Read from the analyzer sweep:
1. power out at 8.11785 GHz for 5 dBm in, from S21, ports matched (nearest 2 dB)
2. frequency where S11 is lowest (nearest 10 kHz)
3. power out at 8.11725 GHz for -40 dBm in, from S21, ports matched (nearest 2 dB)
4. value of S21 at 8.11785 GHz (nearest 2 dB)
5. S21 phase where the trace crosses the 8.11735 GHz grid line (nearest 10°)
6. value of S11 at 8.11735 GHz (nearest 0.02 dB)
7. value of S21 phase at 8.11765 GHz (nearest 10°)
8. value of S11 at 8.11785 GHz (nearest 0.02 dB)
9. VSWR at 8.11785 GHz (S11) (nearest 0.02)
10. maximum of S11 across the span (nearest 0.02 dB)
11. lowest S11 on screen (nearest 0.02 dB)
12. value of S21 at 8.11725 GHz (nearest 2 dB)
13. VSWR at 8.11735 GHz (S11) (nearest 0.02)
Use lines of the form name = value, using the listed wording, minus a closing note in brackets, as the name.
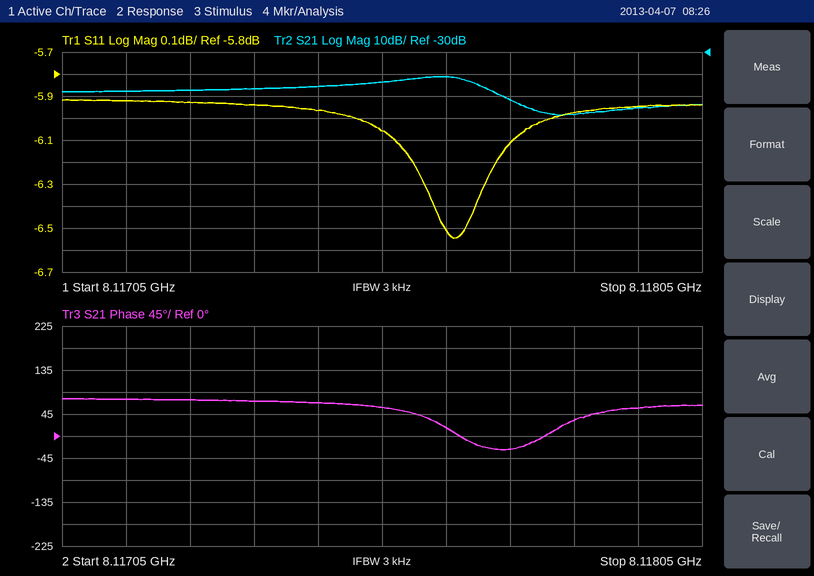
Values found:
power out at 8.11785 GHz for 5 dBm in, from S21, ports matched = -54 dBm
frequency where S11 is lowest = 8.11766 GHz
power out at 8.11725 GHz for -40 dBm in, from S21, ports matched = -88 dBm
value of S21 at 8.11785 GHz = -58 dB
S21 phase where the trace crosses the 8.11735 GHz grid line = 70°
value of S11 at 8.11735 GHz = -5.94 dB
value of S21 phase at 8.11765 GHz = 20°
value of S11 at 8.11785 GHz = -5.98 dB
VSWR at 8.11785 GHz (S11) = 3.02
maximum of S11 across the span = -5.92 dB
lowest S11 on screen = -6.54 dB
value of S21 at 8.11725 GHz = -48 dB
VSWR at 8.11735 GHz (S11) = 3.04
